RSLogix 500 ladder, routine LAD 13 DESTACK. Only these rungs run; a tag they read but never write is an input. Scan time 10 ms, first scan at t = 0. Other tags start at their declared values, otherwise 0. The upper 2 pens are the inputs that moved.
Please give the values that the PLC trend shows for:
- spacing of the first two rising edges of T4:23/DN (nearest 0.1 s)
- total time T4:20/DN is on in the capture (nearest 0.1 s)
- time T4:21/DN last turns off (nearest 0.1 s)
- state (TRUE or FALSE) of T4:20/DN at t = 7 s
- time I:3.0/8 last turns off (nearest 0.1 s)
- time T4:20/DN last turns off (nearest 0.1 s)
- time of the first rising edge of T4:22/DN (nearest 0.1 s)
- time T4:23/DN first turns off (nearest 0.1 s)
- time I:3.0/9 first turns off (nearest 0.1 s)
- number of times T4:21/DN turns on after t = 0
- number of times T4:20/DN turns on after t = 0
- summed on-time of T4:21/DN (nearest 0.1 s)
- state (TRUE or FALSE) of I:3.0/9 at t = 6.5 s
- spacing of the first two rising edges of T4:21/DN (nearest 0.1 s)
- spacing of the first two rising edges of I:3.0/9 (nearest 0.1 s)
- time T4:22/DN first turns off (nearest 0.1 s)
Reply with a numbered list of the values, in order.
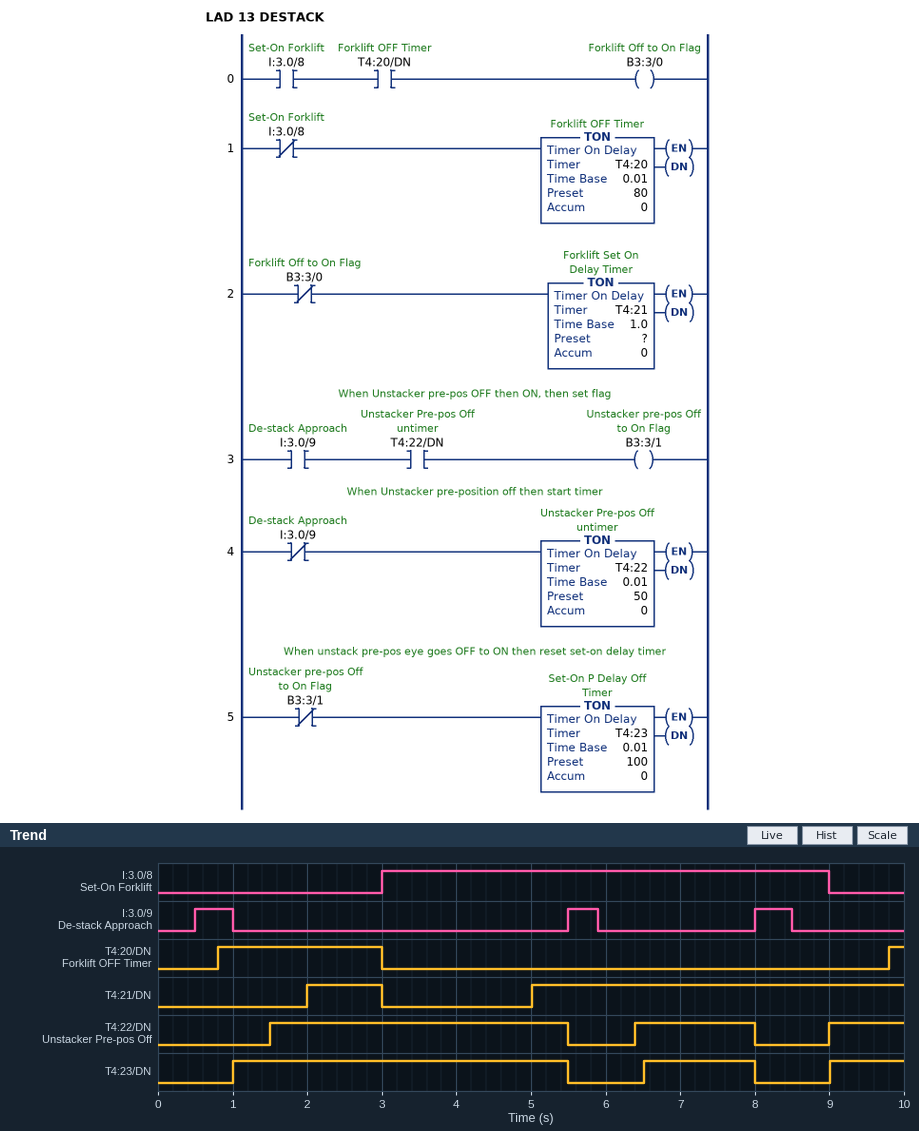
1. 5.5 s
2. 2.4 s
3. 3.0 s
4. FALSE
5. 9.0 s
6. 3.0 s
7. 1.5 s
8. 5.5 s
9. 1.0 s
10. 2
11. 2
12. 6.0 s
13. FALSE
14. 3.0 s
15. 5.0 s
16. 5.5 s
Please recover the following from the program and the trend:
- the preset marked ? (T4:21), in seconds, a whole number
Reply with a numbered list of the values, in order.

1. 2 s
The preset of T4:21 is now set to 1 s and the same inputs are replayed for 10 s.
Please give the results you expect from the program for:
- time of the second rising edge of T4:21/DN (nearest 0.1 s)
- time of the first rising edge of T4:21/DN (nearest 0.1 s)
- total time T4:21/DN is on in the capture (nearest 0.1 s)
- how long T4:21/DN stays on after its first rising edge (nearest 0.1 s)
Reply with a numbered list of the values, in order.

1. 4.0 s
2. 1.0 s
3. 8.0 s
4. 2.0 s
